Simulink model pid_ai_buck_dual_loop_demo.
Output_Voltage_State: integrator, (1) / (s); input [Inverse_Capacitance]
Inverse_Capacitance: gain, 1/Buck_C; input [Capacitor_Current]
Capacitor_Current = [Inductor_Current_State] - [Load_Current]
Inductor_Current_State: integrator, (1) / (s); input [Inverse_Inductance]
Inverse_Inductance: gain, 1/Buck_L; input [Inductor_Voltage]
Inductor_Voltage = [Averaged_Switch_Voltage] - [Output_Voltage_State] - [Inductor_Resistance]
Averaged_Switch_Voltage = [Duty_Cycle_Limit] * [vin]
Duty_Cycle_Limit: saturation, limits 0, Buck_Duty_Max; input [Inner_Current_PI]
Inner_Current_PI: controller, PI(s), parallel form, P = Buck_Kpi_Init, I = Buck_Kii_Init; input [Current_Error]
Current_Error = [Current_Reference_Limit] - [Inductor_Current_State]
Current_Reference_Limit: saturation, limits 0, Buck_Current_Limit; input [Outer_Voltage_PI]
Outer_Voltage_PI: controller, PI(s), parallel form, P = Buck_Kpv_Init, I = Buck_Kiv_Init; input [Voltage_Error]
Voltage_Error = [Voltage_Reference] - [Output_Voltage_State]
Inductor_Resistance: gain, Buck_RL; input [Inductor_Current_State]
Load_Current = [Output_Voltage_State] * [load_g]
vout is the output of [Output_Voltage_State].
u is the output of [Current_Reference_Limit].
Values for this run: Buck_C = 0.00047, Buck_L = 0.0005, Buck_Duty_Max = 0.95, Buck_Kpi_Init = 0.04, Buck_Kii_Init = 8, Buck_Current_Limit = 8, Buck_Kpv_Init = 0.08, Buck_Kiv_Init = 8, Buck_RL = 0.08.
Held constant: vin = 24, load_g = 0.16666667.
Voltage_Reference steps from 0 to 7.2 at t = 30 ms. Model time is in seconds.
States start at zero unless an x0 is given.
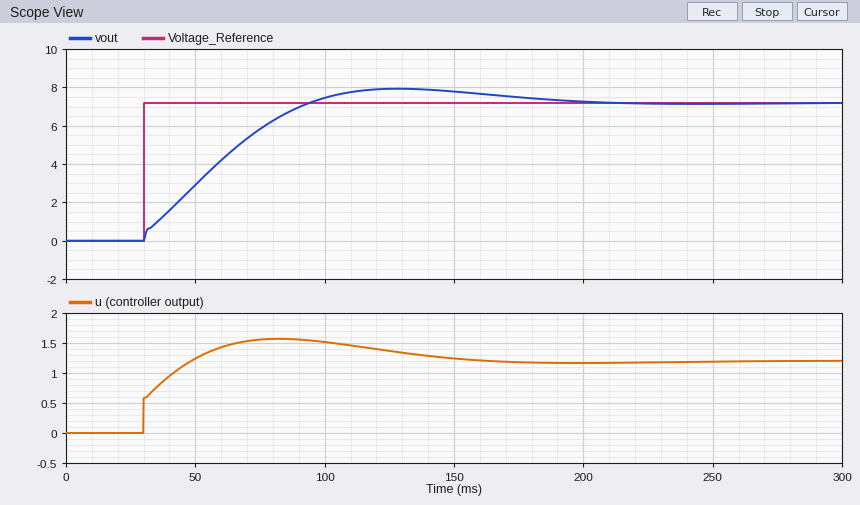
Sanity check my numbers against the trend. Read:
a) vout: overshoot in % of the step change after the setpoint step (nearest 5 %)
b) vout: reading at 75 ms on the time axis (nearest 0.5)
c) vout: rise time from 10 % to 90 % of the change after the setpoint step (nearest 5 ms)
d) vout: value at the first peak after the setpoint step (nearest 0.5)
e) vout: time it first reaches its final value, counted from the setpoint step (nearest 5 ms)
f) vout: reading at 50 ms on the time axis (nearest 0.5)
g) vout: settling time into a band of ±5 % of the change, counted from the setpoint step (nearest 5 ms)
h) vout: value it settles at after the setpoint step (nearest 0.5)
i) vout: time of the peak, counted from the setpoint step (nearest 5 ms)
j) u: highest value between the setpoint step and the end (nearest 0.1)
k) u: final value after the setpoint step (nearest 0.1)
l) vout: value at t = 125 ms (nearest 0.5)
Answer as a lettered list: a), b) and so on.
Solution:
a) 10 %
b) 6.0
c) 50 ms
d) 8.0
e) 65 ms
f) 3.0
g) 140 ms
h) 7.0
i) 100 ms
j) 1.6
k) 1.2
l) 8.0
